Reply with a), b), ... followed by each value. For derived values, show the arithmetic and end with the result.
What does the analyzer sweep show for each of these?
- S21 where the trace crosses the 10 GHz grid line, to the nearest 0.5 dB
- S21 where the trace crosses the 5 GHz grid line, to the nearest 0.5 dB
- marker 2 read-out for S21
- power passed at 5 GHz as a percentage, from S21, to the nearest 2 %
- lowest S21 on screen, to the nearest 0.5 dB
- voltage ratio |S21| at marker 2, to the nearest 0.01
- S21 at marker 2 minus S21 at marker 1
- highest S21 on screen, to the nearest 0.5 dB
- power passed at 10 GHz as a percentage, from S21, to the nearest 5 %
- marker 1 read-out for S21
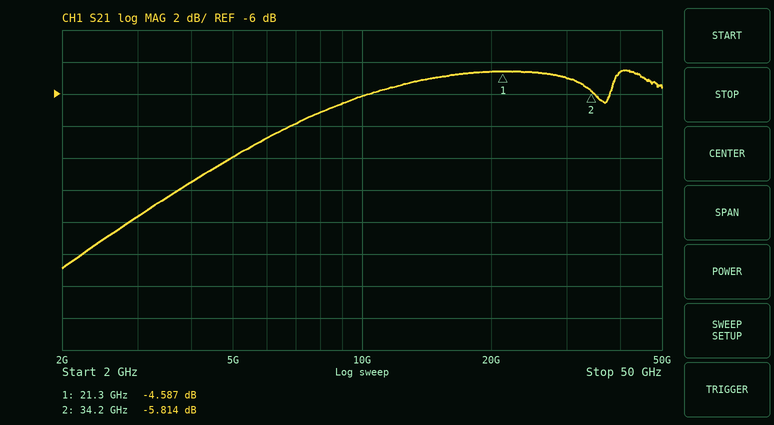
a) -6.0 dB
b) -10.0 dB
c) -5.814 dB
d) 10^(-10/10) ≈ 10 %
e) -17.0 dB
f) 10^(-5.814/20) ≈ 0.51
g) -5.814 − (-4.587) = -1.227 dB
h) -4.5 dB
i) 10^(-6/10) ≈ 25 %
j) -4.587 dB
